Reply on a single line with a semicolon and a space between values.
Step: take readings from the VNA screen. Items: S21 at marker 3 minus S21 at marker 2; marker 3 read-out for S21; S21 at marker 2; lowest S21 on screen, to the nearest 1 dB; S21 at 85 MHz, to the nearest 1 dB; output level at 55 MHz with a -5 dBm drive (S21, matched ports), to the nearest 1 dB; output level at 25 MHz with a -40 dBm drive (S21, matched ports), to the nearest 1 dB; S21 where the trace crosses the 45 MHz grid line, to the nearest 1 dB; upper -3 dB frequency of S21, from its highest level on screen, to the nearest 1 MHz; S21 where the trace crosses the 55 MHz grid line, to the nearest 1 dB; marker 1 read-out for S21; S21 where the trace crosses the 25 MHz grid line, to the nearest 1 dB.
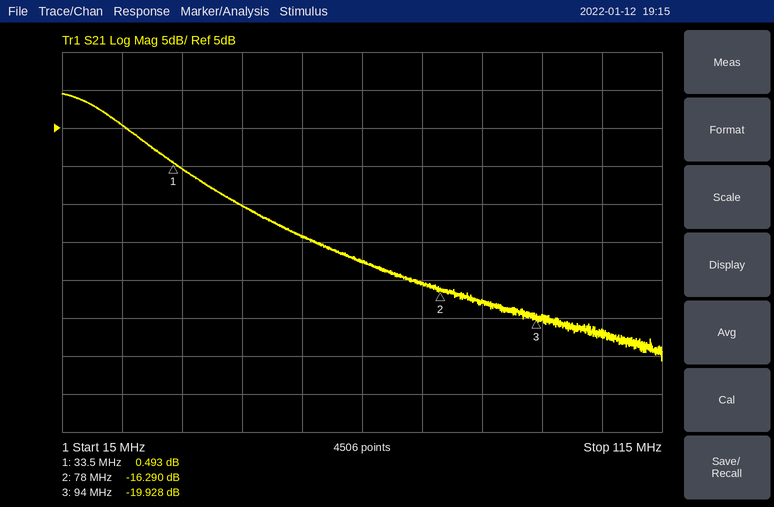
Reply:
-3.638 dB; -19.928 dB; -16.290 dB; -26 dB; -18 dB; -14 dBm; -35 dBm; -5 dB; 23 MHz; -9 dB; 0.493 dB; 5 dB
